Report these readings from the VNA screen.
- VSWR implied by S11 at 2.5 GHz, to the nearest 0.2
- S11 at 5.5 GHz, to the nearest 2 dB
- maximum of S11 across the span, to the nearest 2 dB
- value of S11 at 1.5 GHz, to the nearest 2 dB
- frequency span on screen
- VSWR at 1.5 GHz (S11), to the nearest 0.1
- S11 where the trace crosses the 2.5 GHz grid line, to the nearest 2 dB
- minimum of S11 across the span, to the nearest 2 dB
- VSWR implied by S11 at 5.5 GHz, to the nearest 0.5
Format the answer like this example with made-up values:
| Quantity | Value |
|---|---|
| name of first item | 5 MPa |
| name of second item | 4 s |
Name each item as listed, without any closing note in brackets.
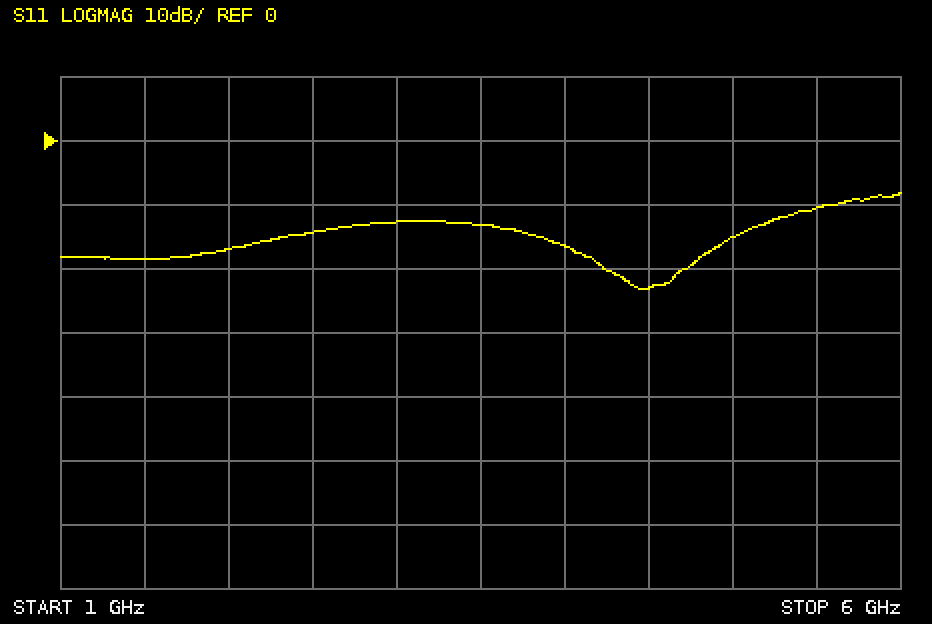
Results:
| Quantity | Value |
|---|---|
| VSWR implied by S11 at 2.5 GHz, to the nearest 0.2 | 1.4 |
| S11 at 5.5 GHz, to the nearest 2 dB | -10 dB |
| maximum of S11 across the span, to the nearest 2 dB | -8 dB |
| value of S11 at 1.5 GHz, to the nearest 2 dB | -18 dB |
| frequency span on screen | 5 GHz |
| VSWR at 1.5 GHz (S11), to the nearest 0.1 | 1.3 |
| S11 where the trace crosses the 2.5 GHz grid line, to the nearest 2 dB | -14 dB |
| minimum of S11 across the span, to the nearest 2 dB | -24 dB |
| VSWR implied by S11 at 5.5 GHz, to the nearest 0.5 | 2.0 |
